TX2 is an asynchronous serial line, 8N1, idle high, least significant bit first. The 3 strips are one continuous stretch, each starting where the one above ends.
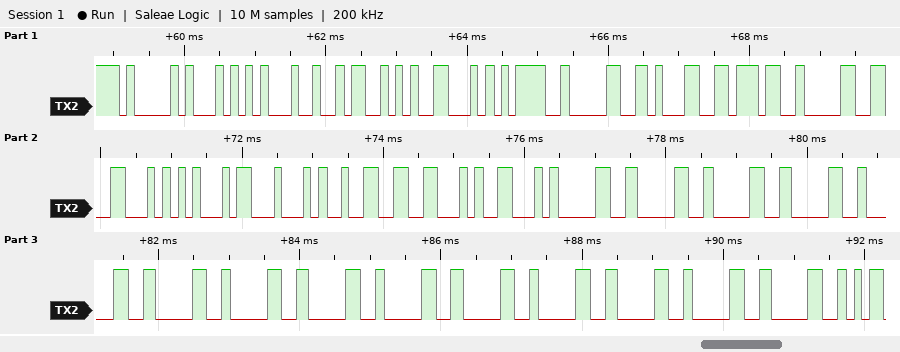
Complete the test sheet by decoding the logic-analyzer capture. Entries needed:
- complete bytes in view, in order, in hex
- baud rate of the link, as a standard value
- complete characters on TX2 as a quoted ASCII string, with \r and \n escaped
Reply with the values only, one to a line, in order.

41 54 24 53 46 3D 30 31 37 30 46 45 44 32 46 46 30 30 30 30 30 30 30 30 30 30 30 30 30 30
9600 baud
"AT$SF=0170FED2FF00000000000000"
